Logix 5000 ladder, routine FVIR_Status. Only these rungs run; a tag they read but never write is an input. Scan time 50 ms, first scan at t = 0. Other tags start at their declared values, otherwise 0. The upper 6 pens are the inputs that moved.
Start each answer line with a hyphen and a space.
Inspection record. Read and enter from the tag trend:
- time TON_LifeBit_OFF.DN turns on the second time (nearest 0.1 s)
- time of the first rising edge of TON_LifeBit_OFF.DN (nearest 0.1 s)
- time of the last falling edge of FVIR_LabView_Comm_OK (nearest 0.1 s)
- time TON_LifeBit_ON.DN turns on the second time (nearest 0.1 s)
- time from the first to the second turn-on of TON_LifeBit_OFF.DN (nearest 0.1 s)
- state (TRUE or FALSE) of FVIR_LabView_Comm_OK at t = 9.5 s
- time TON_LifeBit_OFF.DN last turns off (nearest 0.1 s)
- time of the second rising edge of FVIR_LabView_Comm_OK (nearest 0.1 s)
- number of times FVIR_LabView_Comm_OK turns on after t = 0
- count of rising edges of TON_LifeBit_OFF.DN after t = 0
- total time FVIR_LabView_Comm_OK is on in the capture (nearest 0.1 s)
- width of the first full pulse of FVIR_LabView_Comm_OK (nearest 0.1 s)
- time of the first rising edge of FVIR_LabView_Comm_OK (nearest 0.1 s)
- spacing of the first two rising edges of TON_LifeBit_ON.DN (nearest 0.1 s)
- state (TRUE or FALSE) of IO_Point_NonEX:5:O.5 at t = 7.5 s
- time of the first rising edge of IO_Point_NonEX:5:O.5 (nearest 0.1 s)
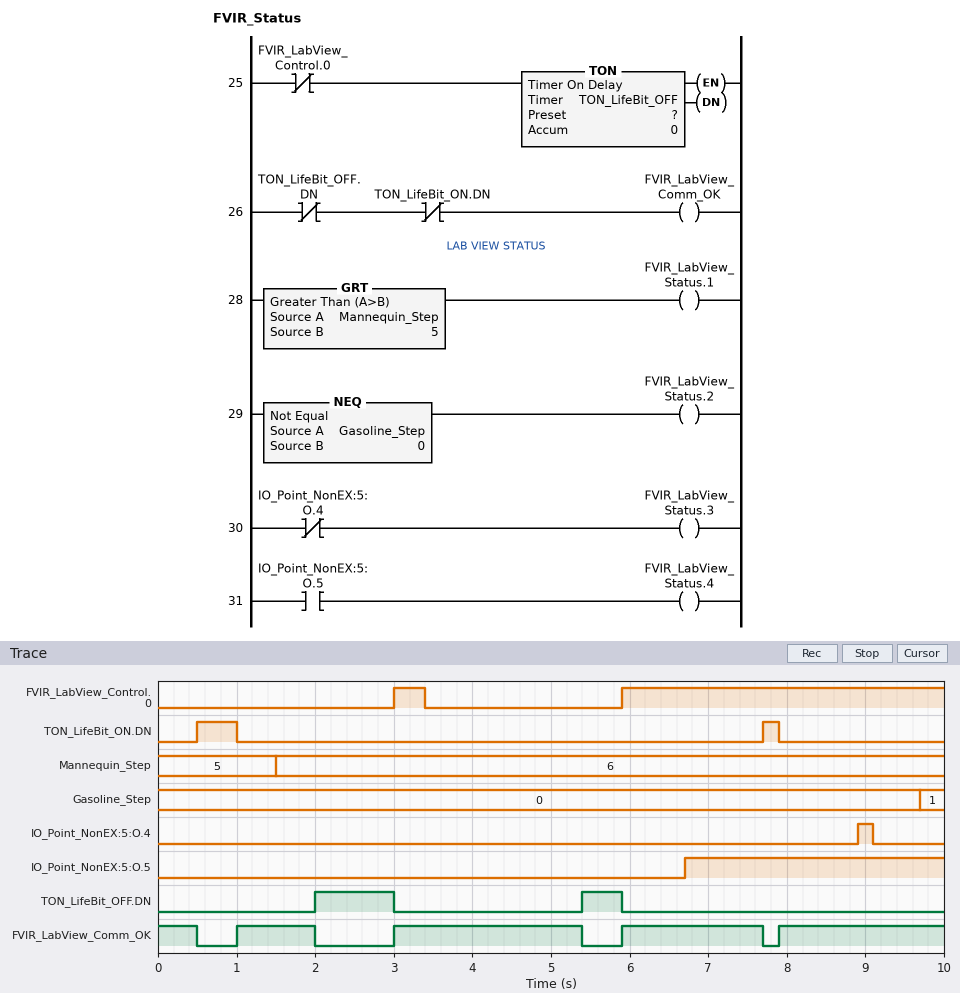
- 5.4 s
- 2.0 s
- 7.7 s
- 7.7 s
- 3.4 s
- TRUE
- 5.9 s
- 3.0 s
- 4
- 2
- 7.8 s
- 1.0 s
- 1.0 s
- 7.2 s
- TRUE
- 6.7 s
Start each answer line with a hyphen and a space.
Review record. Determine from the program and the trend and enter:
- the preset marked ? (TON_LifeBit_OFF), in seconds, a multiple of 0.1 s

- 2.0 s
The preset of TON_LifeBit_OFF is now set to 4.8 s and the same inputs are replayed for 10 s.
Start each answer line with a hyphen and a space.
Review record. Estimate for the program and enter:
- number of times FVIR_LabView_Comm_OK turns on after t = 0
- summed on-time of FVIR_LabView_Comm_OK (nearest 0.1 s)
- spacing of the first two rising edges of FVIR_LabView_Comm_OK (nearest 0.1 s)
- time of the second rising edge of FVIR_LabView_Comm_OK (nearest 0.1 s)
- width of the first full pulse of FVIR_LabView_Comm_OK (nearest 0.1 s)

- 2
- 9.3 s
- 6.9 s
- 7.9 s
- 6.7 s
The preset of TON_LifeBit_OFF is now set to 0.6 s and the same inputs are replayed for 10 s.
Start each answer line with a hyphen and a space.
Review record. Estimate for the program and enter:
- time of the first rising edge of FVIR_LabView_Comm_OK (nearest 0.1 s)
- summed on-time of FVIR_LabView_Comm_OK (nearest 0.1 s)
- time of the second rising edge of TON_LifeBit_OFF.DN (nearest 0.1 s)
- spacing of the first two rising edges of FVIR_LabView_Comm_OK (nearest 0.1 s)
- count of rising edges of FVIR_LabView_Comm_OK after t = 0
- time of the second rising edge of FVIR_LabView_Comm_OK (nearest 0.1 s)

- 3.0 s
- 5.4 s
- 4.0 s
- 2.9 s
- 3
- 5.9 s
